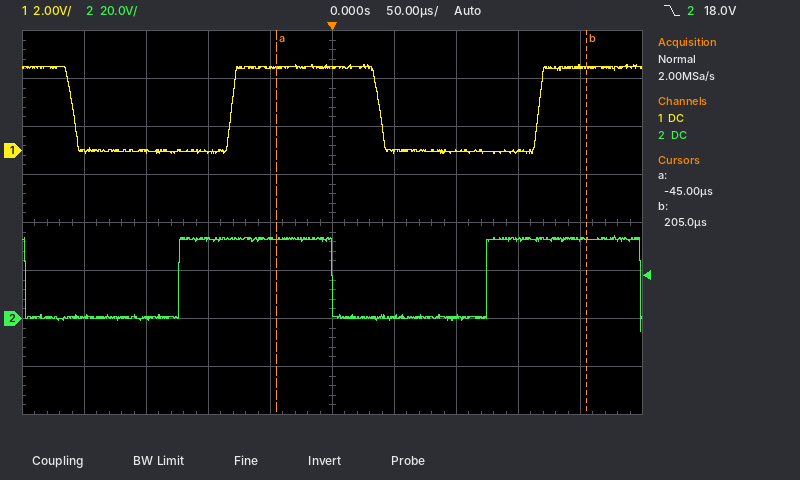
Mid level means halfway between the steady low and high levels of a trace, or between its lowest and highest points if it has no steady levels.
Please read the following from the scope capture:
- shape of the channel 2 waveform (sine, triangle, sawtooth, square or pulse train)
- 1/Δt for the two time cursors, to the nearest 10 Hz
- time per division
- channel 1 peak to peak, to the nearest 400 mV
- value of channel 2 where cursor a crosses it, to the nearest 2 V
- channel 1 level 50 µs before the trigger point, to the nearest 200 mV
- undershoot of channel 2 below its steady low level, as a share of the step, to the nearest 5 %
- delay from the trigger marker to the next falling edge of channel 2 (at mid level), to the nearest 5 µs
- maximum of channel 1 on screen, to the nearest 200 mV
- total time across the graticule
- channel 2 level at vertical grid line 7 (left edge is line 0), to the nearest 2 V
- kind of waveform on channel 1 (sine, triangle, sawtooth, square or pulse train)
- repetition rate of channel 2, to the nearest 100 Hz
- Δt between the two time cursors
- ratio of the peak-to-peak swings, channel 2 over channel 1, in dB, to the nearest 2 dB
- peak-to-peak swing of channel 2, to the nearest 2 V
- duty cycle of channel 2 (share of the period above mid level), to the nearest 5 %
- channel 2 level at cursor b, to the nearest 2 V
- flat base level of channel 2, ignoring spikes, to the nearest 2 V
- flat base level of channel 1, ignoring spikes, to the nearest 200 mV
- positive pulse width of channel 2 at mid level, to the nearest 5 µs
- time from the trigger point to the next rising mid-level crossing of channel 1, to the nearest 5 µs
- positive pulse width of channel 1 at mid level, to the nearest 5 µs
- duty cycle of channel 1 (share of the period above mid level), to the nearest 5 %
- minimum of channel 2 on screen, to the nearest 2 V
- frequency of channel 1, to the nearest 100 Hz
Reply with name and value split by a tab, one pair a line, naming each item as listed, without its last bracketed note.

shape of the channel 2 waveform	square
1/Δt for the two time cursors, to the nearest 10 Hz	4.00 kHz
time per division	50 µs
channel 1 peak to peak, to the nearest 400 mV	3.6 V
value of channel 2 where cursor a crosses it, to the nearest 2 V	34 V
channel 1 level 50 µs before the trigger point, to the nearest 200 mV	3.4 V
undershoot of channel 2 below its steady low level, as a share of the step, to the nearest 5 %	20 %
delay from the trigger marker to the next falling edge of channel 2 (at mid level), to the nearest 5 µs	250 µs
maximum of channel 1 on screen, to the nearest 200 mV	3.6 V
total time across the graticule	500 µs
channel 2 level at vertical grid line 7 (left edge is line 0), to the nearest 2 V	0 V
kind of waveform on channel 1	square
repetition rate of channel 2, to the nearest 100 Hz	4.0 kHz
Δt between the two time cursors	250 µs
ratio of the peak-to-peak swings, channel 2 over channel 1, in dB, to the nearest 2 dB	20 dB
peak-to-peak swing of channel 2, to the nearest 2 V	40 V
duty cycle of channel 2 (share of the period above mid level), to the nearest 5 %	50 %
channel 2 level at cursor b, to the nearest 2 V	34 V
flat base level of channel 2, ignoring spikes, to the nearest 2 V	0 V
flat base level of channel 1, ignoring spikes, to the nearest 200 mV	0.0 V
positive pulse width of channel 2 at mid level, to the nearest 5 µs	125 µs
time from the trigger point to the next rising mid-level crossing of channel 1, to the nearest 5 µs	165 µs
positive pulse width of channel 1 at mid level, to the nearest 5 µs	120 µs
duty cycle of channel 1 (share of the period above mid level), to the nearest 5 %	50 %
minimum of channel 2 on screen, to the nearest 2 V	-6 V
frequency of channel 1, to the nearest 100 Hz	4.0 kHz
